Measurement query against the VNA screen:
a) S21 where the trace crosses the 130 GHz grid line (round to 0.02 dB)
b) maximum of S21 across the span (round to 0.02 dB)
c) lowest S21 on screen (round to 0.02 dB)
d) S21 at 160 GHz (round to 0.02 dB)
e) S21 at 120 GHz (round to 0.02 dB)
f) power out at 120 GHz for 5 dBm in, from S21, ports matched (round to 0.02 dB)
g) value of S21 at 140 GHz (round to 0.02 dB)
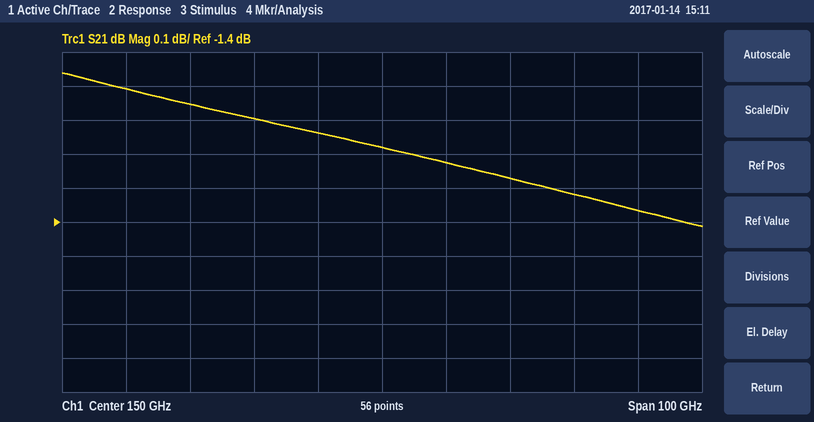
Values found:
-1.10 dB
-0.96 dB
-1.42 dB
-1.22 dB
-1.06 dB
3.94 dBm
-1.14 dB
